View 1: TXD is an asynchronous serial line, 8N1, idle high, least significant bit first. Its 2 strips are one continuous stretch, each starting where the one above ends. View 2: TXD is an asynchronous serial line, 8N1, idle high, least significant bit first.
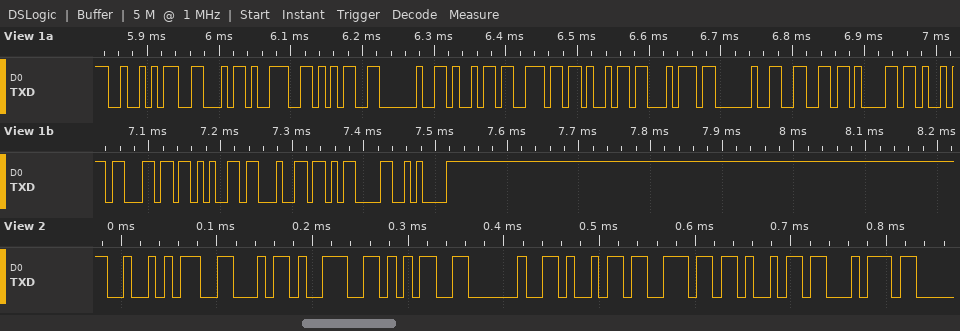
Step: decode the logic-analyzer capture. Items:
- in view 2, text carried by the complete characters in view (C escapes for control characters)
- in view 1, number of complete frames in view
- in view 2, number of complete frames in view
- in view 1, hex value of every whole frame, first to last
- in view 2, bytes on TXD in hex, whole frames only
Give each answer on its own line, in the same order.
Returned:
"RF95 init"
18
9
52 46 39 35 20 69 6E 69 74 20 66 61 69 6C 65 64 0D 0A
52 46 39 35 20 69 6E 69 74
